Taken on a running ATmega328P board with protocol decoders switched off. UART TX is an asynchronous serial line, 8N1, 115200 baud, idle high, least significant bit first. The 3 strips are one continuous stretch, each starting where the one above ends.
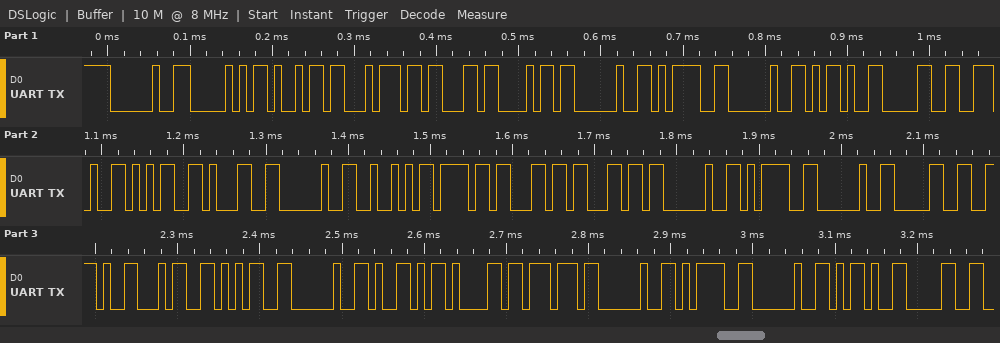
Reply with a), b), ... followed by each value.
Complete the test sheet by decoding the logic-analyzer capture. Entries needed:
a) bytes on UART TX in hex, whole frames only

a) 0x20 0x50 0x69 0x74 0x63 0x68 0x20 0x3D 0x20 0x2D 0x30 0x2E 0x35 0x31 0x20 0x52 0x6F 0x6C 0x6C 0x20 0x3D 0x20 0x30 0x2E 0x34 0x35 0x20 0x59 0x61 0x77 0x20 0x3D 0x20 0x2D 0x30
